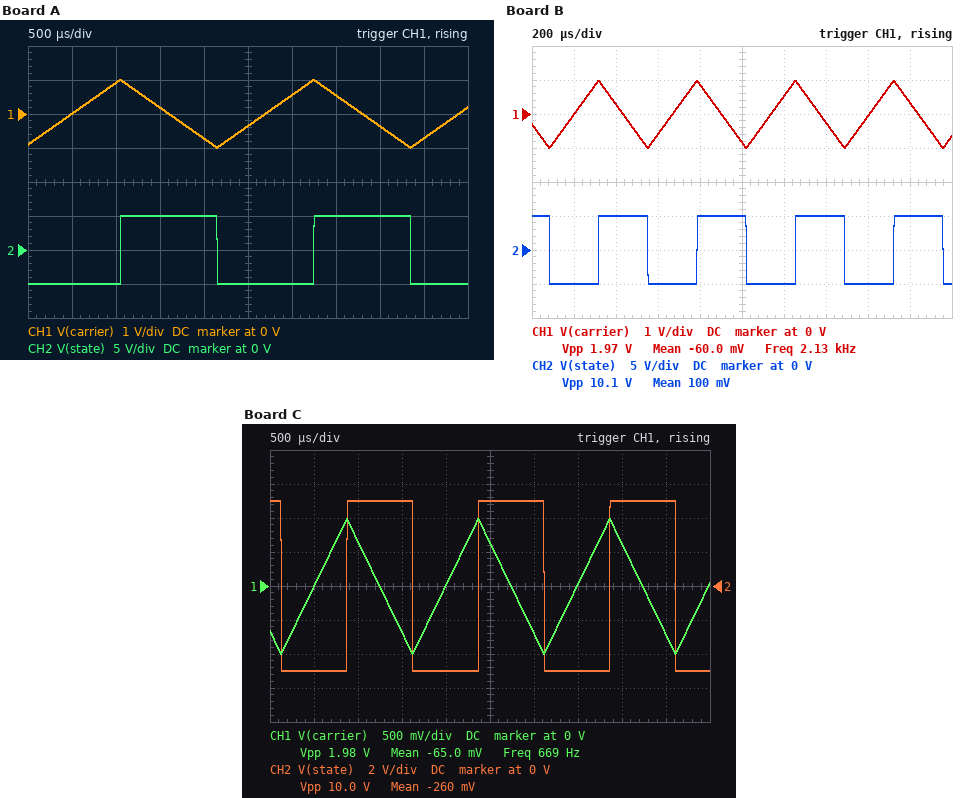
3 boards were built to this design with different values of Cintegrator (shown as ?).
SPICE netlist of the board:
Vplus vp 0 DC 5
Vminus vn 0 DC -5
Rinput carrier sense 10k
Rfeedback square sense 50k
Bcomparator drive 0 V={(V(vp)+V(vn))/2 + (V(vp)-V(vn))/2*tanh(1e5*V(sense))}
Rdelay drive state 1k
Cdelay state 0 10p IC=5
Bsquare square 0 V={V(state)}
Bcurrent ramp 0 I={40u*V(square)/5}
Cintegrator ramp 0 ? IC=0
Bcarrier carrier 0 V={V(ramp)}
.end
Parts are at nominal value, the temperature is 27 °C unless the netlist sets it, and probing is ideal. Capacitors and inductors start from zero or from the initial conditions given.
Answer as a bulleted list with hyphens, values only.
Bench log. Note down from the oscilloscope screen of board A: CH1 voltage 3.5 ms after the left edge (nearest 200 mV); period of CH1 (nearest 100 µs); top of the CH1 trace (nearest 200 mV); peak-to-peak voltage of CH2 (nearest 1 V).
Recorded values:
- 600 mV
- 2.2 ms
- 1.0 V
- 10 V
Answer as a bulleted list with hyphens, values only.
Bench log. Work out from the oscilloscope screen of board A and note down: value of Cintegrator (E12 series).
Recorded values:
- 22 nF
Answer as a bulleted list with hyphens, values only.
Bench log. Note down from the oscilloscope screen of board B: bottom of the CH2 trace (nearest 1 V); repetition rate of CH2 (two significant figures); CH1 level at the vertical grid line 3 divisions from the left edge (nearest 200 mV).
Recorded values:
- -5 V
- 2.1 kHz
- -600 mV
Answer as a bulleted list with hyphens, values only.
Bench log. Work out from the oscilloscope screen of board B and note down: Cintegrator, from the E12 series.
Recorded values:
- 4.7 nF
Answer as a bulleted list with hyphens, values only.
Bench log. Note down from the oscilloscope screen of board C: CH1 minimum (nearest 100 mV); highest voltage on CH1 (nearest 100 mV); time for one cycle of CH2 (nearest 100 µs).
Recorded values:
- -1.0 V
- 1.0 V
- 1.5 ms
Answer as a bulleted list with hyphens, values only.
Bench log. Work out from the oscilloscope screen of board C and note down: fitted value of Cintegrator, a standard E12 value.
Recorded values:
- 15 nF
